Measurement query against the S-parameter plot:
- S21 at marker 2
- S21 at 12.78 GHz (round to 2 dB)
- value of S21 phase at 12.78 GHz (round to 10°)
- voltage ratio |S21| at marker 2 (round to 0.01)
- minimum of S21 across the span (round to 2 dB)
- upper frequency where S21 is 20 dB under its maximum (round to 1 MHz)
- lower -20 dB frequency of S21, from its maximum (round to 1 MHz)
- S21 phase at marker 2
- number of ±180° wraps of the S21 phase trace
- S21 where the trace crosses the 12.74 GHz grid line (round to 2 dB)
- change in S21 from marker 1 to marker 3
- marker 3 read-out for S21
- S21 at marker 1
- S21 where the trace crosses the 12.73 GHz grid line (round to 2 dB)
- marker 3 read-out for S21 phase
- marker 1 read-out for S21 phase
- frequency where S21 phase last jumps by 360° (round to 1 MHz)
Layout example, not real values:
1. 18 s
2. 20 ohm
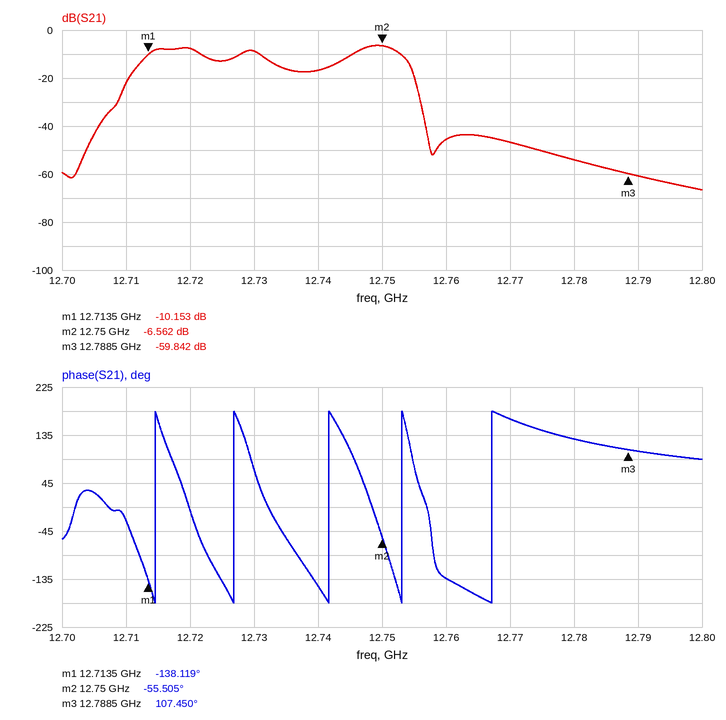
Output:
1. -6.562 dB
2. -54 dB
3. 130°
4. 0.47
5. -66 dB
6. 12.756 GHz
7. 12.709 GHz
8. -55.505°
9. 5
10. -16 dB
11. -49.689 dB
12. -59.842 dB
13. -10.153 dB
14. -8 dB
15. 107.450°
16. -138.119°
17. 12.767 GHz
